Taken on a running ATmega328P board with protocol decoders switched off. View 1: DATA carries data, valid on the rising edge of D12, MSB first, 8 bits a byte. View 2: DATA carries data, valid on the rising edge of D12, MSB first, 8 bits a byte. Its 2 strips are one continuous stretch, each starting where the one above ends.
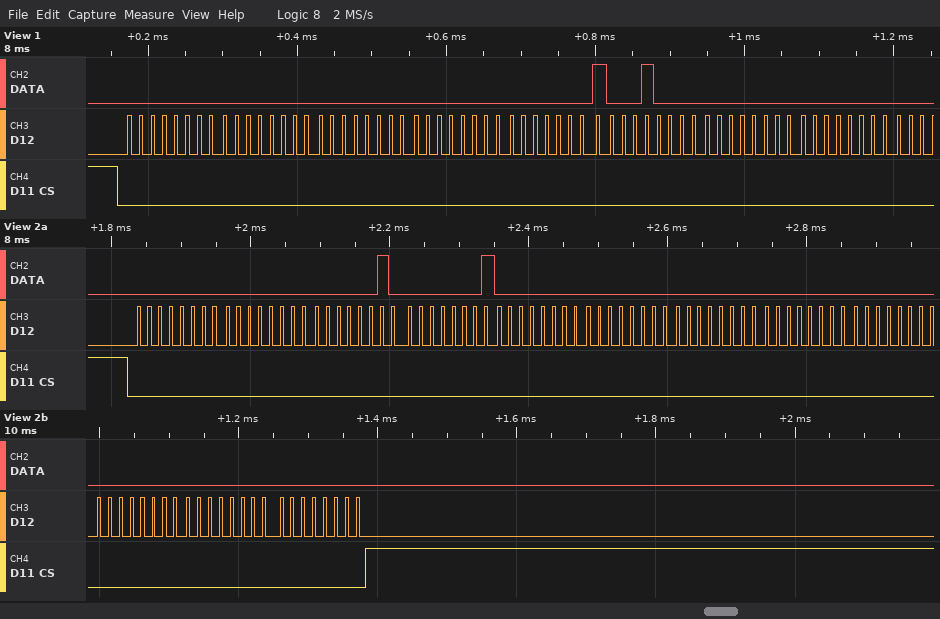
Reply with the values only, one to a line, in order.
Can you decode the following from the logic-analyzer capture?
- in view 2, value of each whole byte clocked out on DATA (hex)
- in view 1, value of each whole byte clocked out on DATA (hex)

0x00 0x00 0x02 0x01 0x00 0x00 0x00 0x00 0x00 0x00 0x00 0x00
00 00 00 00 01 10 00 00
